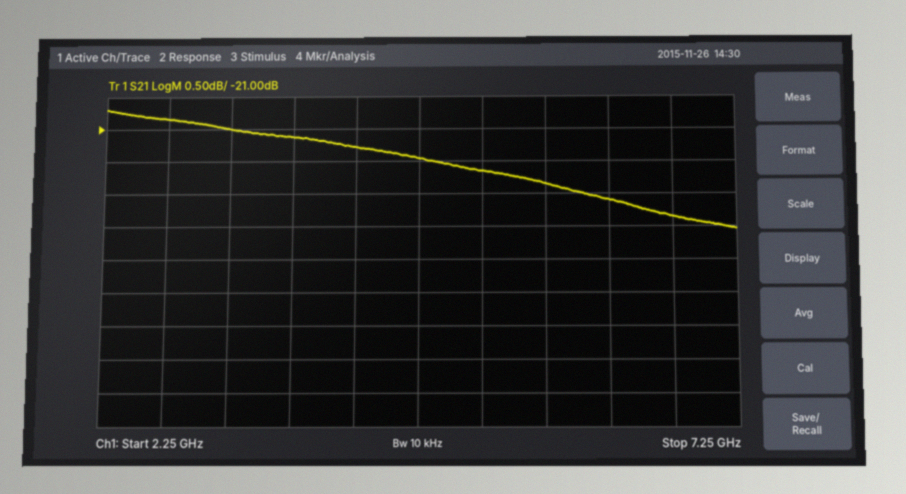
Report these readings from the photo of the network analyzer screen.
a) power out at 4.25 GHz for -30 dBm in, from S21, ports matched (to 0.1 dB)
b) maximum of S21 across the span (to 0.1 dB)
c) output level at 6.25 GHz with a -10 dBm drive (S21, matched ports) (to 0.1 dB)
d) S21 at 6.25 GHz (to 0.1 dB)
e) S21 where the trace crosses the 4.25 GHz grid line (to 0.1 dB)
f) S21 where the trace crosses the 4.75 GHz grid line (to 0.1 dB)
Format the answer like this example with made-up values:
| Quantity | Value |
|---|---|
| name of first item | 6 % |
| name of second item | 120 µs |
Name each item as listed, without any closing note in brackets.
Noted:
| Quantity | Value |
|---|---|
| power out at 4.25 GHz for -30 dBm in, from S21, ports matched | -51.3 dBm |
| maximum of S21 across the span | -20.7 dB |
| output level at 6.25 GHz with a -10 dBm drive (S21, matched ports) | -32.1 dBm |
| S21 at 6.25 GHz | -22.1 dB |
| S21 where the trace crosses the 4.25 GHz grid line | -21.3 dB |
| S21 where the trace crosses the 4.75 GHz grid line | -21.5 dB |
